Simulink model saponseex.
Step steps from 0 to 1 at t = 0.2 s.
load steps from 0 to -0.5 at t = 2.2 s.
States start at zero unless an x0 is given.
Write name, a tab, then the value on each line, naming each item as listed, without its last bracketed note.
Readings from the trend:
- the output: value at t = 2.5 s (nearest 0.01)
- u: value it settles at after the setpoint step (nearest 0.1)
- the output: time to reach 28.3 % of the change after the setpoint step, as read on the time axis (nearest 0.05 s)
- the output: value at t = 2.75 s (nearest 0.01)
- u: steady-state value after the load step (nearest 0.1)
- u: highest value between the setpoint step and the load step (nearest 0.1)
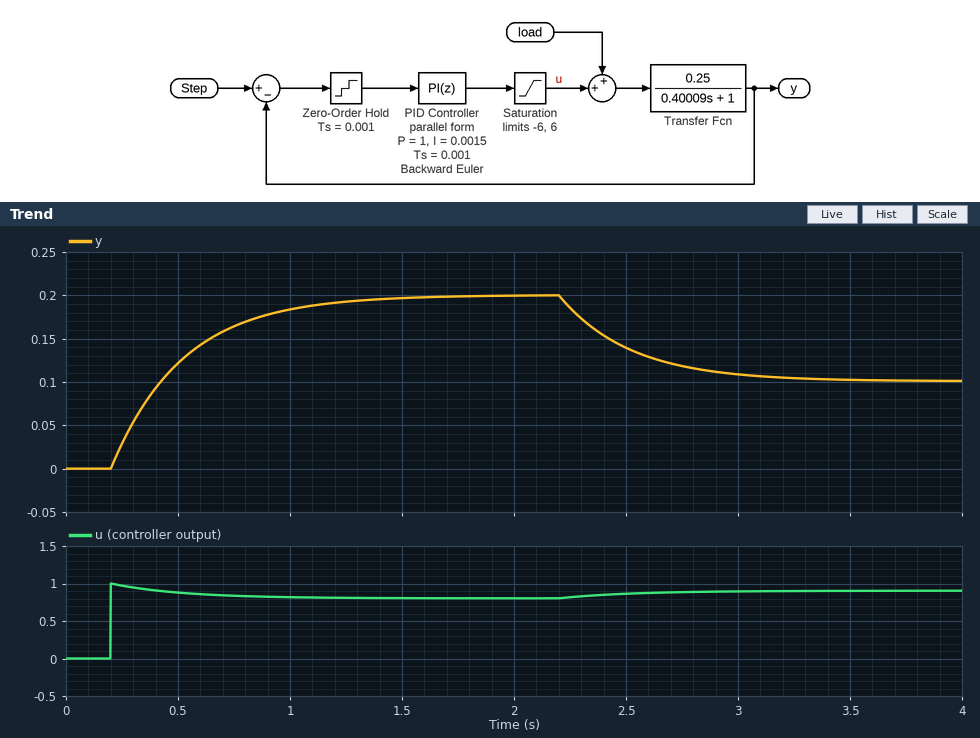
the output: value at t = 2.5 s	0.14
u: value it settles at after the setpoint step	0.8
the output: time to reach 28.3 % of the change after the setpoint step, as read on the time axis	0.30 s
the output: value at t = 2.75 s	0.12
u: steady-state value after the load step	0.9
u: highest value between the setpoint step and the load step	1.0
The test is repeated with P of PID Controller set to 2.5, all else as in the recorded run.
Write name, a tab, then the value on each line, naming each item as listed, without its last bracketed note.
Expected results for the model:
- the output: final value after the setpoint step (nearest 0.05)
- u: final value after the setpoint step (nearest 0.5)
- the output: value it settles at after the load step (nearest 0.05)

the output: final value after the setpoint step	0.40
u: final value after the setpoint step	1.5
the output: value it settles at after the load step	0.30
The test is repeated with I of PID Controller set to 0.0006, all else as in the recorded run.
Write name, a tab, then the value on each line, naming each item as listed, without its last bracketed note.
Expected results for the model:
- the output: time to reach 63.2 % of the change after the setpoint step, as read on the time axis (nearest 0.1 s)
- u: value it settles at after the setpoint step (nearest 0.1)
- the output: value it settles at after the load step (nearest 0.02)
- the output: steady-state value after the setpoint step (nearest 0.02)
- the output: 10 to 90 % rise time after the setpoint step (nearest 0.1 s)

the output: time to reach 63.2 % of the change after the setpoint step, as read on the time axis	0.5 s
u: value it settles at after the setpoint step	0.8
the output: value it settles at after the load step	0.10
the output: steady-state value after the setpoint step	0.20
the output: 10 to 90 % rise time after the setpoint step	0.7 s
